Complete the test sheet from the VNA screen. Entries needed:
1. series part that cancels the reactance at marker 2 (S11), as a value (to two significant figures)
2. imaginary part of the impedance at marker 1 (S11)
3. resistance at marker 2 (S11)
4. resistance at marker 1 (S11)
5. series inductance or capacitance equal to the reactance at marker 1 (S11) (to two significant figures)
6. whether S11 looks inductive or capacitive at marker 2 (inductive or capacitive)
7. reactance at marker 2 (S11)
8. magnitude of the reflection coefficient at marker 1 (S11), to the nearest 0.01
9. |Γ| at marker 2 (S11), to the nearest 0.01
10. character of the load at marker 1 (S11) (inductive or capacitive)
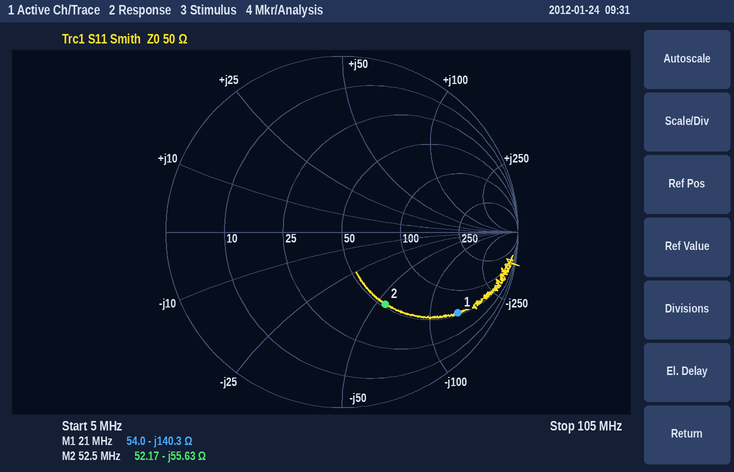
170 nH
-140.3 Ω
52.17 Ω
54.0 Ω
54 pF
capacitive
-55.63 Ω
0.80
0.48
capacitive
